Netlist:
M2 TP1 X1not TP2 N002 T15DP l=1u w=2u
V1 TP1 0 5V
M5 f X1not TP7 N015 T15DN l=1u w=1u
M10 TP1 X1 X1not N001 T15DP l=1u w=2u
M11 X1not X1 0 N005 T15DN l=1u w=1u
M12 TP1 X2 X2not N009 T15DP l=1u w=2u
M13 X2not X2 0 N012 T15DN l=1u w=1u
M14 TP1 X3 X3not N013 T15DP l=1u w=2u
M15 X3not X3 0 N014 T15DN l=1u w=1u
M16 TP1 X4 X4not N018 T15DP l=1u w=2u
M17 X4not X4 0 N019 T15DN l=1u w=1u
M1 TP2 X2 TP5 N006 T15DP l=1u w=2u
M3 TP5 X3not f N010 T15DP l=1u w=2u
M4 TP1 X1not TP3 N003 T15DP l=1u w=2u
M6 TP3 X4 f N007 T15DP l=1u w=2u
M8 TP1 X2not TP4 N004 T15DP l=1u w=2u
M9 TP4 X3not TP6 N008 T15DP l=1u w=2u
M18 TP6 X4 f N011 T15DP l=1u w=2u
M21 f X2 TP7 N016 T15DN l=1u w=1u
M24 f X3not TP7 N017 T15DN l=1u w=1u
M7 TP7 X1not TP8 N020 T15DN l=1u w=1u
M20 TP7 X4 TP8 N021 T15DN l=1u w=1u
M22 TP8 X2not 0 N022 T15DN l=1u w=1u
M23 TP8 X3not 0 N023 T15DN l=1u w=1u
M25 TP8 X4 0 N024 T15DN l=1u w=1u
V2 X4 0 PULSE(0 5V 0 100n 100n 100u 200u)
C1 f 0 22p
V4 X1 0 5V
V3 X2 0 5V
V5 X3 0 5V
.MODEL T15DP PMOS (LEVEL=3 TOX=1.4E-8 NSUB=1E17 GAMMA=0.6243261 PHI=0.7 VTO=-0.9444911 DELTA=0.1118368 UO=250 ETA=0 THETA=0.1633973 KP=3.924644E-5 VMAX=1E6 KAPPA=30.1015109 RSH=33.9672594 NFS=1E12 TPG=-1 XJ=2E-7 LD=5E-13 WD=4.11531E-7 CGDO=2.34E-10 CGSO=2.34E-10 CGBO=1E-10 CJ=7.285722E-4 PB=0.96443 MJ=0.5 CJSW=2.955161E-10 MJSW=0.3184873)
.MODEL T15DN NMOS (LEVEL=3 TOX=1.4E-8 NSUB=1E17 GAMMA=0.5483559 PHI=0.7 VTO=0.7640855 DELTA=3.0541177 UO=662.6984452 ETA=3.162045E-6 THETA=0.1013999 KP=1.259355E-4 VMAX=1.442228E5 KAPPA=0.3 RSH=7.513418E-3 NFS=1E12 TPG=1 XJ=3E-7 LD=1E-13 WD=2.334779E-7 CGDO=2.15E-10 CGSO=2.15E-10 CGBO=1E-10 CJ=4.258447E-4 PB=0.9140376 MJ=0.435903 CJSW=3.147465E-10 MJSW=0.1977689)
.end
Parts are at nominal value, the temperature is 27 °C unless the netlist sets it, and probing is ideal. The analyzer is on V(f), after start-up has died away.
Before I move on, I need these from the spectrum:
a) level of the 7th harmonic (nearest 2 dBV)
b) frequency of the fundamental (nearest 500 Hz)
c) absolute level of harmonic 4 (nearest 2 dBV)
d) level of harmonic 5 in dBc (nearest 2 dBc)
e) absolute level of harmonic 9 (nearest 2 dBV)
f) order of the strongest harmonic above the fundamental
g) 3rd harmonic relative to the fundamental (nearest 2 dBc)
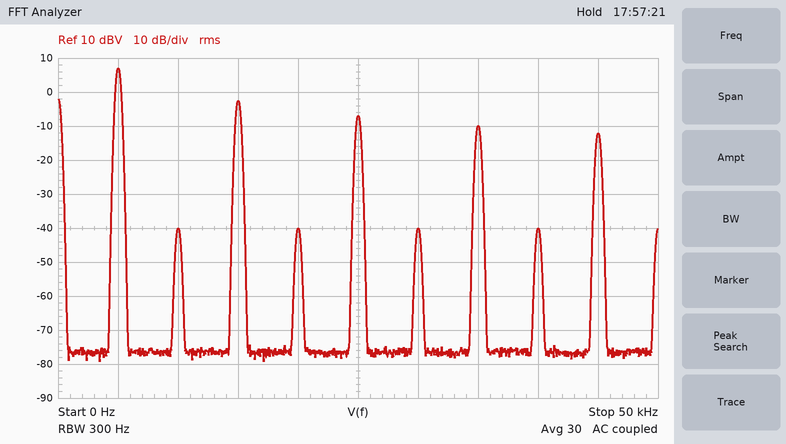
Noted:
-10 dBV
5.0 kHz
-40 dBV
-14 dBc
-12 dBV
3
-10 dBc
